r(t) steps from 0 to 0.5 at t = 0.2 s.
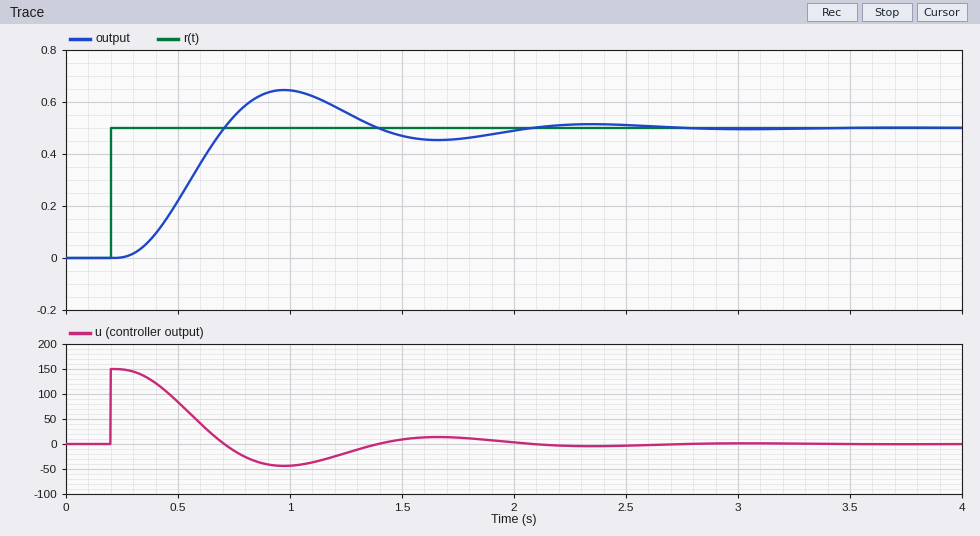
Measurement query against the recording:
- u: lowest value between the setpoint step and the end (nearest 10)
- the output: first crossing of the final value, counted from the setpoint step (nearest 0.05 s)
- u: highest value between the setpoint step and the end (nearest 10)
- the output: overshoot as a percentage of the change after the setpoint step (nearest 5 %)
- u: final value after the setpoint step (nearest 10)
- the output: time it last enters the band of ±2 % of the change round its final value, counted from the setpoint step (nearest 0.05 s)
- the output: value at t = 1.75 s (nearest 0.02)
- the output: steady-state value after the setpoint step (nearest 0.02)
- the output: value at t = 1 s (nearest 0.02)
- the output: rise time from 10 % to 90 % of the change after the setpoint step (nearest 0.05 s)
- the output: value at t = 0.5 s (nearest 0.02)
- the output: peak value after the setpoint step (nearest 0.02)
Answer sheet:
-40
0.50 s
150
30 %
0
2.35 s
0.46
0.50
0.64
0.30 s
0.22
0.64
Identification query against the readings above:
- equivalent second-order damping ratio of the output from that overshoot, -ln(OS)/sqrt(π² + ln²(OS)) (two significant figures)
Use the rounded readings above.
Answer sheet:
0.36
